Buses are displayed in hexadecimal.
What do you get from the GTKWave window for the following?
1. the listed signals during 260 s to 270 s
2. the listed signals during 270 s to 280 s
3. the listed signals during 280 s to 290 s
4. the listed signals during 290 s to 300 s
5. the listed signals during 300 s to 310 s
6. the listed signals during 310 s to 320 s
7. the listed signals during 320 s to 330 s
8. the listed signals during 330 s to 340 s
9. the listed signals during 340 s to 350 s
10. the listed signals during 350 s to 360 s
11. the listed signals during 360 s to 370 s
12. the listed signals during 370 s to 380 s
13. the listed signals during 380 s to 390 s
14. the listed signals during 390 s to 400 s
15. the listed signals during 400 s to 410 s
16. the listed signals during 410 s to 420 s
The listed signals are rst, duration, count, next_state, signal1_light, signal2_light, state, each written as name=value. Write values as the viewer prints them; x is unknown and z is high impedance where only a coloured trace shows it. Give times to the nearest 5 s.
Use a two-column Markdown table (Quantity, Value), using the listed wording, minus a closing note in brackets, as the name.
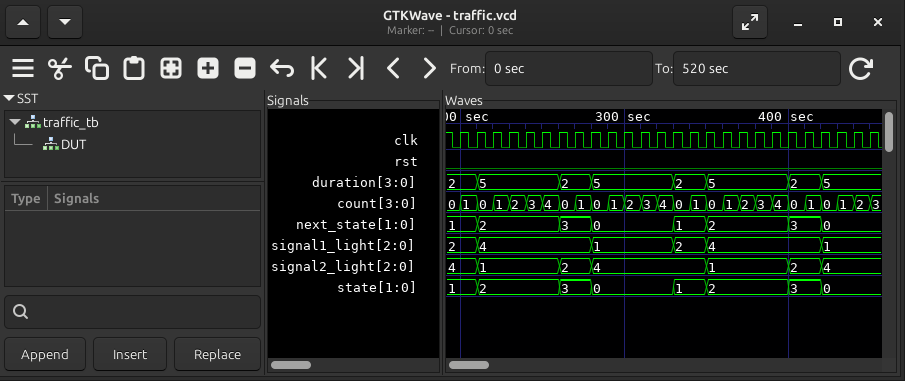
| Quantity | Value |
|---|---|
| the listed signals during 260 s to 270 s | rst=0, duration=2, count=0, next_state=3, signal1_light=4, signal2_light=2, state=3 |
| the listed signals during 270 s to 280 s | rst=0, duration=2, count=1, next_state=3, signal1_light=4, signal2_light=2, state=3 |
| the listed signals during 280 s to 290 s | rst=0, duration=5, count=0, next_state=0, signal1_light=1, signal2_light=4, state=0 |
| the listed signals during 290 s to 300 s | rst=0, duration=5, count=1, next_state=0, signal1_light=1, signal2_light=4, state=0 |
| the listed signals during 300 s to 310 s | rst=0, duration=5, count=2, next_state=0, signal1_light=1, signal2_light=4, state=0 |
| the listed signals during 310 s to 320 s | rst=0, duration=5, count=3, next_state=0, signal1_light=1, signal2_light=4, state=0 |
| the listed signals during 320 s to 330 s | rst=0, duration=5, count=4, next_state=0, signal1_light=1, signal2_light=4, state=0 |
| the listed signals during 330 s to 340 s | rst=0, duration=2, count=0, next_state=1, signal1_light=2, signal2_light=4, state=1 |
| the listed signals during 340 s to 350 s | rst=0, duration=2, count=1, next_state=1, signal1_light=2, signal2_light=4, state=1 |
| the listed signals during 350 s to 360 s | rst=0, duration=5, count=0, next_state=2, signal1_light=4, signal2_light=1, state=2 |
| the listed signals during 360 s to 370 s | rst=0, duration=5, count=1, next_state=2, signal1_light=4, signal2_light=1, state=2 |
| the listed signals during 370 s to 380 s | rst=0, duration=5, count=2, next_state=2, signal1_light=4, signal2_light=1, state=2 |
| the listed signals during 380 s to 390 s | rst=0, duration=5, count=3, next_state=2, signal1_light=4, signal2_light=1, state=2 |
| the listed signals during 390 s to 400 s | rst=0, duration=5, count=4, next_state=2, signal1_light=4, signal2_light=1, state=2 |
| the listed signals during 400 s to 410 s | rst=0, duration=2, count=0, next_state=3, signal1_light=4, signal2_light=2, state=3 |
| the listed signals during 410 s to 420 s | rst=0, duration=2, count=1, next_state=3, signal1_light=4, signal2_light=2, state=3 |
